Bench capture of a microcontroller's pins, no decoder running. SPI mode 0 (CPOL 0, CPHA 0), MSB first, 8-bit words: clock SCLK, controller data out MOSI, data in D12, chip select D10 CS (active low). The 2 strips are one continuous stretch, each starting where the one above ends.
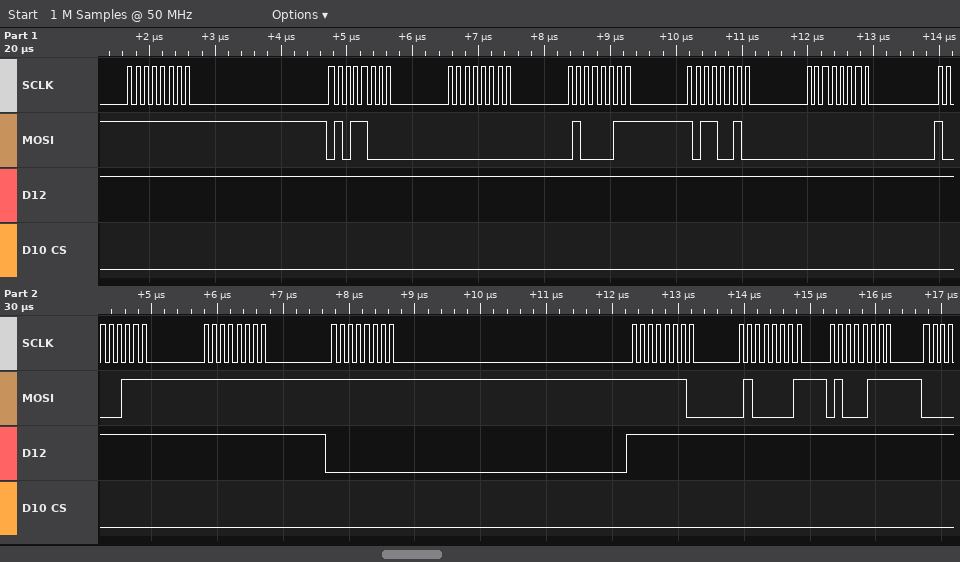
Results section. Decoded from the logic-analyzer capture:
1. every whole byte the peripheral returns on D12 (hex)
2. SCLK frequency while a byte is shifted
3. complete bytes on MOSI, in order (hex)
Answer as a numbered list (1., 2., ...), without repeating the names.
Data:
1. FF FF FF FF FF FF FF FF 00 FF FF FF
2. 8 MHz
3. FF 58 00 43 B2 00 87 FF FF FE 41 47
